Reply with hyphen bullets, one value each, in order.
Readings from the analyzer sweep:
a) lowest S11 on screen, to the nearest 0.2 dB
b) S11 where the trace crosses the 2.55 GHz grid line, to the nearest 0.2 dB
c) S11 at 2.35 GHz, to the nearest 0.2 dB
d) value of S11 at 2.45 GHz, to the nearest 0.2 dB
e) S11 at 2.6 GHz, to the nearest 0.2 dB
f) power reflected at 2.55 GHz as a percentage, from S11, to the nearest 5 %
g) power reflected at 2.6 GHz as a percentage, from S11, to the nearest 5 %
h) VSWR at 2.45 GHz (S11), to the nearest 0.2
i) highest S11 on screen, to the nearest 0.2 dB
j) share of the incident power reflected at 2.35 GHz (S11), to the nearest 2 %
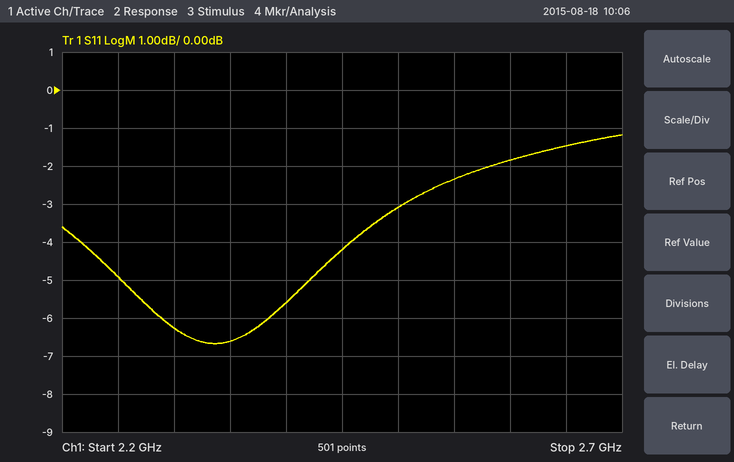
- -6.6 dB
- -2.4 dB
- -6.6 dB
- -4.2 dB
- -1.8 dB
- 60 %
- 65 %
- 4.2
- -1.2 dB
- 22 %
